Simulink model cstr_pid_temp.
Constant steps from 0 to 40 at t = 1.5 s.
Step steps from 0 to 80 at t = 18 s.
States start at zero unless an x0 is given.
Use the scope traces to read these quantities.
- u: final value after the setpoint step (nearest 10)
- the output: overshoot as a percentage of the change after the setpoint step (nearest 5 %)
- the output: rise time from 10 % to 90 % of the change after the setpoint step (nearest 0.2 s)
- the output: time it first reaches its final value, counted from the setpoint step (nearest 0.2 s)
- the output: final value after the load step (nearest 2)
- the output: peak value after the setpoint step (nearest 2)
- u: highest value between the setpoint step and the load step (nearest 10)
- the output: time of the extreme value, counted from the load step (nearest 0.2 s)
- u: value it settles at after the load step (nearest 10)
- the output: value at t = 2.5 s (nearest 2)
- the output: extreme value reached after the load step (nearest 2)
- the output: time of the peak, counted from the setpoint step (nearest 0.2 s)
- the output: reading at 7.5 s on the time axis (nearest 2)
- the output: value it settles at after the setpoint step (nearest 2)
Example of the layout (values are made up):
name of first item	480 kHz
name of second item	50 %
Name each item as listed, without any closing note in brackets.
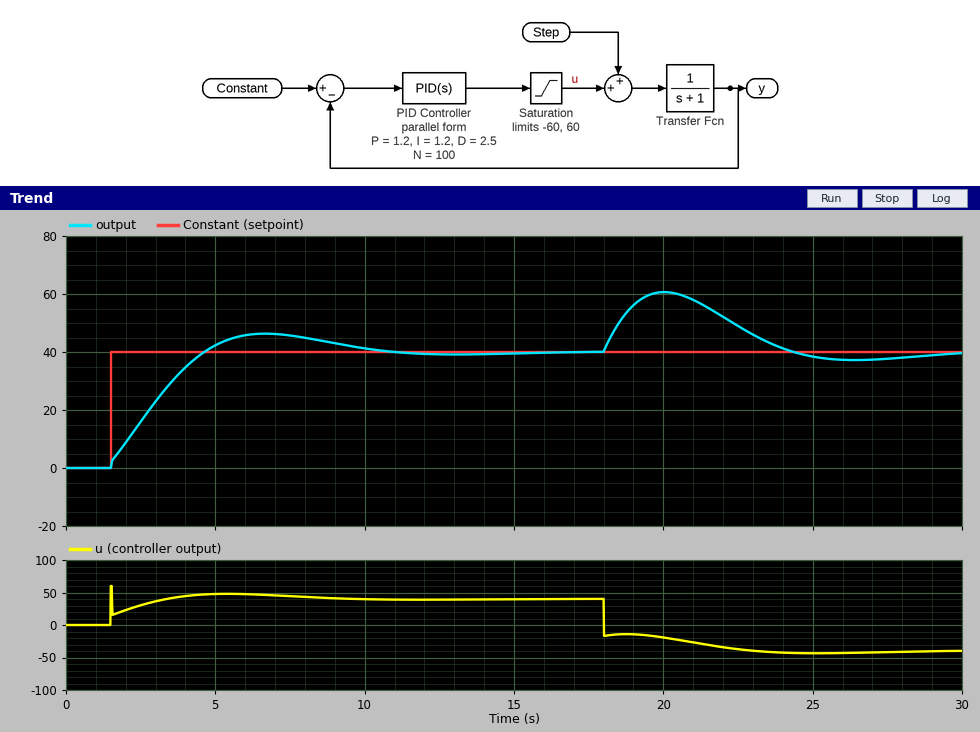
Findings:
u: final value after the setpoint step	40
the output: overshoot as a percentage of the change after the setpoint step	15 %
the output: rise time from 10 % to 90 % of the change after the setpoint step	2.4 s
the output: time it first reaches its final value, counted from the setpoint step	3.2 s
the output: final value after the load step	40
the output: peak value after the setpoint step	46
u: highest value between the setpoint step and the load step	60
the output: time of the extreme value, counted from the load step	2.0 s
u: value it settles at after the load step	-40
the output: value at t = 2.5 s	16
the output: extreme value reached after the load step	60
the output: time of the peak, counted from the setpoint step	5.2 s
the output: reading at 7.5 s on the time axis	46
the output: value it settles at after the setpoint step	40
